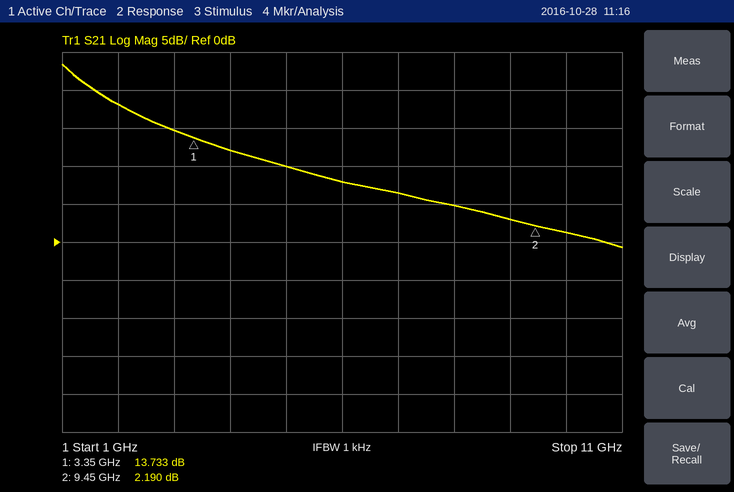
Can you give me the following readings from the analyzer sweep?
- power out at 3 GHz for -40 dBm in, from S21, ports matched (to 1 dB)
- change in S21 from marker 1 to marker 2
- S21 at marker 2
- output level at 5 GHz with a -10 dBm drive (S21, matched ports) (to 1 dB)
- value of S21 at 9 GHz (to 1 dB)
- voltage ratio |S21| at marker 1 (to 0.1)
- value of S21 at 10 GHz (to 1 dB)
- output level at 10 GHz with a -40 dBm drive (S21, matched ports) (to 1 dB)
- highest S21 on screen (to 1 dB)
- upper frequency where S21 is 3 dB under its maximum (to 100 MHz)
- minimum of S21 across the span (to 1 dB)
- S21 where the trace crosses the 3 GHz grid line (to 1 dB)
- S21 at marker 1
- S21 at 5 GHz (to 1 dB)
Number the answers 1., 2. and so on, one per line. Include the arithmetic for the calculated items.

1. -40 dBm + (15 dB) = -25 dBm
2. 2.19 − (13.733) = -11.543 dB
3. 2.190 dB
4. -10 dBm + (10 dB) = 0 dBm
5. 3 dB
6. 10^(13.733/20) ≈ 4.9
7. 1 dB
8. -40 dBm + (1 dB) = -39 dBm
9. 23 dB
10. 1.5 GHz
11. -1 dB
12. 15 dB
13. 13.733 dB
14. 10 dB
